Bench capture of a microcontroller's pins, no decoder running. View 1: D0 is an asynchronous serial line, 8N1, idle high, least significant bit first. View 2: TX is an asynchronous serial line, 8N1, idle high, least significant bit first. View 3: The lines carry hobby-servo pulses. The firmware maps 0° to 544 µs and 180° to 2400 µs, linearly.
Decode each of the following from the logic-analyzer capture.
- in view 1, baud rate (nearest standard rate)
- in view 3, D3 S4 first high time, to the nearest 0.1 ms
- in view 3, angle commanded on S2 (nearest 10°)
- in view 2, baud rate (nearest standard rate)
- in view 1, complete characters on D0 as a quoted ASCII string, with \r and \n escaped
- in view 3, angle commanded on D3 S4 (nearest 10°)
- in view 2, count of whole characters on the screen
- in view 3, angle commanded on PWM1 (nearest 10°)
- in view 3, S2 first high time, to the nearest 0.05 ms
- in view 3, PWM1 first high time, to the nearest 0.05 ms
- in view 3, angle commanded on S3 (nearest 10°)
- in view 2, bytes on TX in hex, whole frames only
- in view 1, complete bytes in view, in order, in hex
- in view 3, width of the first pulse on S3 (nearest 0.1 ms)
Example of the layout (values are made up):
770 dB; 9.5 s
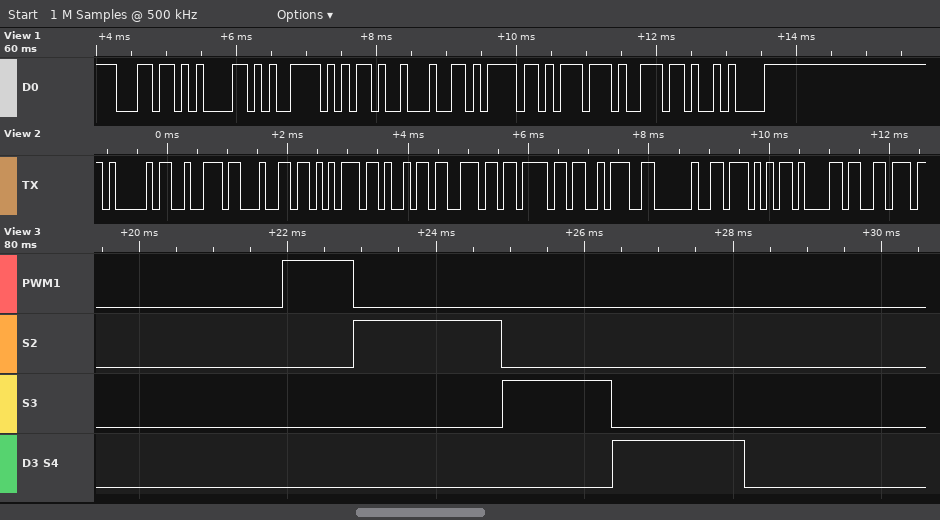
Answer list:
9600 baud; 1.8 ms; 140°; 9600 baud; "lay-down\n"; 120°; 12; 40°; 2.00 ms; 0.95 ms; 90°; 41 72 64 75 69 6E 6F 3A 20 57 61 76; 6C 61 79 2D 64 6F 77 6E 0A; 1.5 ms
